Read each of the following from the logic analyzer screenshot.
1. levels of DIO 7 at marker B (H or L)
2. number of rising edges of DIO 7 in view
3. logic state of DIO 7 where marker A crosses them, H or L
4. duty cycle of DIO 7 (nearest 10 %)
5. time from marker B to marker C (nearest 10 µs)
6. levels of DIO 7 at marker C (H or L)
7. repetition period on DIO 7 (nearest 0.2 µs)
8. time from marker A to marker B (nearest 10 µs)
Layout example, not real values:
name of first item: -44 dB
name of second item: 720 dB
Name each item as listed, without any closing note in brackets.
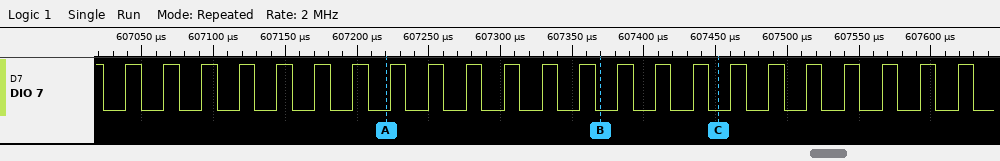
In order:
levels of DIO 7 at marker B: DIO 7=L
number of rising edges of DIO 7 in view: 23
logic state of DIO 7 where marker A crosses them, H or L: DIO 7=L
duty cycle of DIO 7: 40 %
time from marker B to marker C: 80 µs
levels of DIO 7 at marker C: DIO 7=L
repetition period on DIO 7: 26.4 µs
time from marker A to marker B: 150 µs
